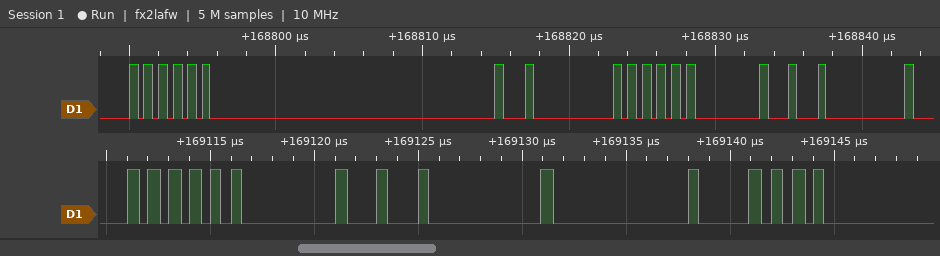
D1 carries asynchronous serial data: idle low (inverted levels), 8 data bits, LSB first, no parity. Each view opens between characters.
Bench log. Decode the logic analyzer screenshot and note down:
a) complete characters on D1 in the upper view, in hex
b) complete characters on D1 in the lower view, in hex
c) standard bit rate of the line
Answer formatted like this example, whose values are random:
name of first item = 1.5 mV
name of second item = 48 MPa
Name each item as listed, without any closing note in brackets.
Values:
complete characters on D1 in the upper view, in hex = 55, FF, F7, 55, FF, 77
complete characters on D1 in the lower view, in hex = 55, FF, 77, FF, 5F, FD
standard bit rate of the line = 2000000 baud
